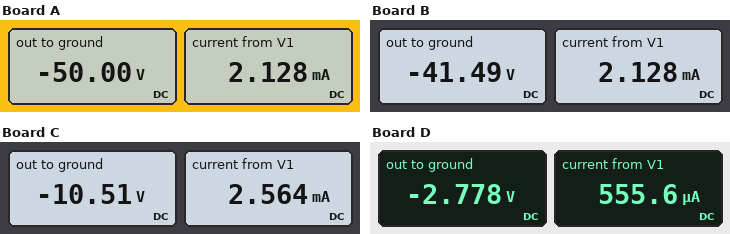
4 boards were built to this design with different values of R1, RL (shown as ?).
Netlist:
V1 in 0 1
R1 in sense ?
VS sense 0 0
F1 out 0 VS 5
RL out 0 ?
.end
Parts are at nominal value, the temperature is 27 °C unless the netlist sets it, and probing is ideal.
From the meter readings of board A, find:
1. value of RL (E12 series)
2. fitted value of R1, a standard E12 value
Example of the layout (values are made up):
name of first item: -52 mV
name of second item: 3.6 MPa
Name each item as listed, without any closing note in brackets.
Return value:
value of RL: 4.7 kΩ
fitted value of R1, a standard E12 value: 470 Ω
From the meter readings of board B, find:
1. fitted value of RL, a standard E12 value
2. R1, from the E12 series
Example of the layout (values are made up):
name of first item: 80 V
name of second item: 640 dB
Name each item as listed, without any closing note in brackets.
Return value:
fitted value of RL, a standard E12 value: 3.9 kΩ
R1, from the E12 series: 470 Ω
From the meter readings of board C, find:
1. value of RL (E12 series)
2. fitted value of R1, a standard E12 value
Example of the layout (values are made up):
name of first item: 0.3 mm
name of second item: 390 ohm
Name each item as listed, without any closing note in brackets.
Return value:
value of RL: 820 Ω
fitted value of R1, a standard E12 value: 390 Ω
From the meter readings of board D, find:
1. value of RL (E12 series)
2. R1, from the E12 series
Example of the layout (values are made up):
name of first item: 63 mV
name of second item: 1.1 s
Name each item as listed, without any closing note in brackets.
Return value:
value of RL: 1 kΩ
R1, from the E12 series: 1.8 kΩ
